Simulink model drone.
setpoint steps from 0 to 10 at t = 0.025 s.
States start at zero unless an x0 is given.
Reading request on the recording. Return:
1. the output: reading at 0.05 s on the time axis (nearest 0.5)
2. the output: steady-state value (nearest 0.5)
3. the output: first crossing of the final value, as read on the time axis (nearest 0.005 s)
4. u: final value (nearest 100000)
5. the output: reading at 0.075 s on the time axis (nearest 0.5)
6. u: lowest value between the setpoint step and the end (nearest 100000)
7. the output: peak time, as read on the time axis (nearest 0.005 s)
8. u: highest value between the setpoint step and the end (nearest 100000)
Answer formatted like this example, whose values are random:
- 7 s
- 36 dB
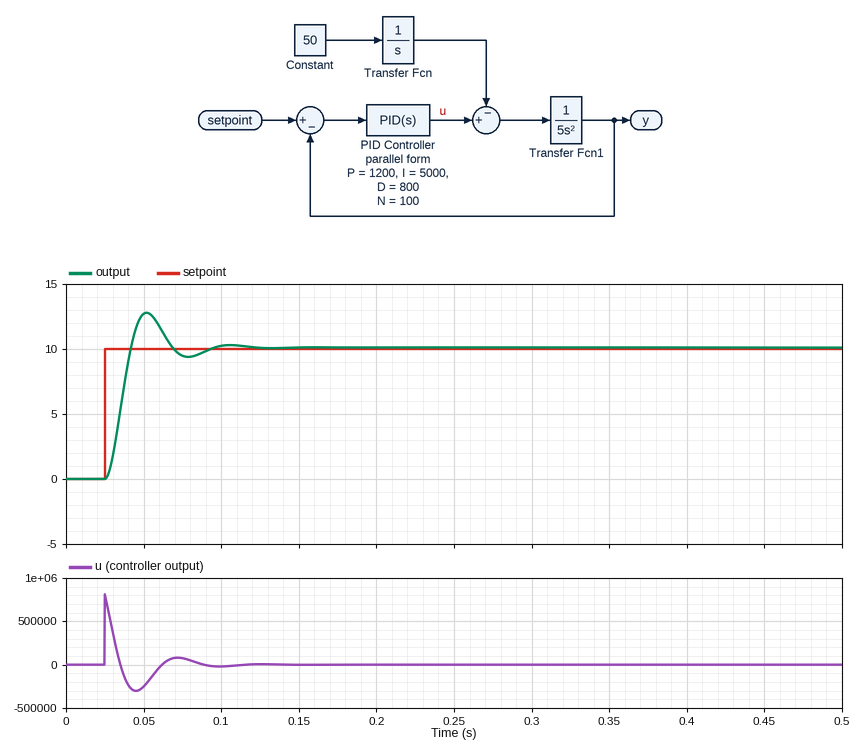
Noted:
- 12.5
- 10.0
- 0.040 s
- 0
- 9.5
- -300000
- 0.050 s
- 800000
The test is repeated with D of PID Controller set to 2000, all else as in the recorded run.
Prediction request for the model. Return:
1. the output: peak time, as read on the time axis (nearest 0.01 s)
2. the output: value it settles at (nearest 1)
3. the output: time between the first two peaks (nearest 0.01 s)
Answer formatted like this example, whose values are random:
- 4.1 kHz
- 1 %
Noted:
- 0.04 s
- 10
- 0.03 s
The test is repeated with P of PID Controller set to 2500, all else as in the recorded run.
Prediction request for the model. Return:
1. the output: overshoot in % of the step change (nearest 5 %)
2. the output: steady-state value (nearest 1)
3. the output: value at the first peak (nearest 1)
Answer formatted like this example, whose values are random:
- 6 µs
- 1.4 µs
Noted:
- 30 %
- 10
- 13
